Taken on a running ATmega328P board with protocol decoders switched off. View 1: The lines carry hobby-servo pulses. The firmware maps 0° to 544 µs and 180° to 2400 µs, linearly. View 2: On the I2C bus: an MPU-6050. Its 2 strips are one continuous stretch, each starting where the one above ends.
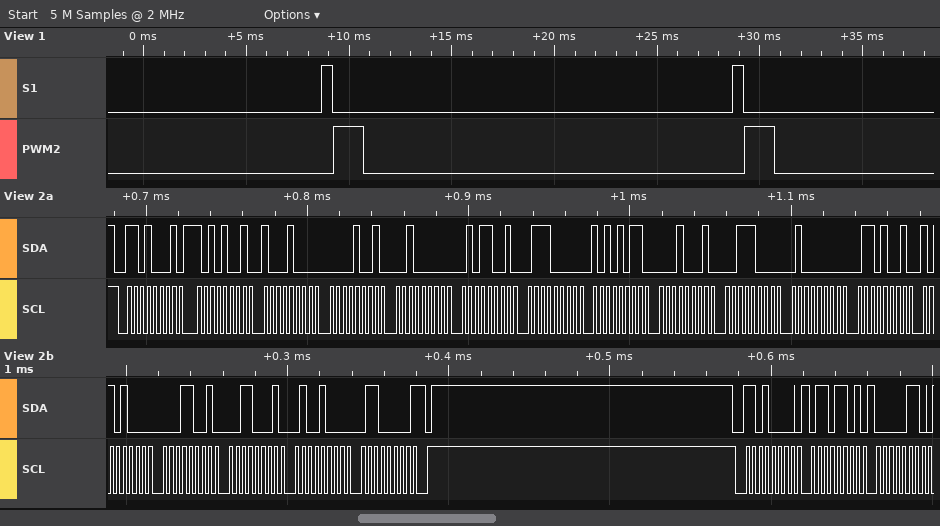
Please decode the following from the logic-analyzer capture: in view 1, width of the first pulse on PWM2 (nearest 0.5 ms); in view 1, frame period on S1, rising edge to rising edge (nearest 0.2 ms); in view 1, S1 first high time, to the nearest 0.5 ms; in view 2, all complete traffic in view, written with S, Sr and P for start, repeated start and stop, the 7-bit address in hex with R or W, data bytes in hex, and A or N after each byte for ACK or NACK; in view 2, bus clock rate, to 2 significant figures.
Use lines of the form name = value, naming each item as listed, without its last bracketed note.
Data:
in view 1, width of the first pulse on PWM2 = 1.5 ms
in view 1, frame period on S1, rising edge to rising edge = 20.0 ms
in view 1, S1 first high time, to the nearest 0.5 ms = 0.5 ms
in view 2, all complete traffic in view, written with S, Sr and P for start, repeated start and stop, the 7-bit address in hex with R or W, data bytes in hex, and A or N after each byte for ACK or NACK = S 68R A A9 A 88 A 09 A 20 A 59 A 70 A AB A 11 A 38 A 40 A 69 A A8 A 19 A 31 A 48 A 60 N P S 68W A 6D A 06 A
in view 2, bus clock rate, to 2 significant figures = 250 kHz
